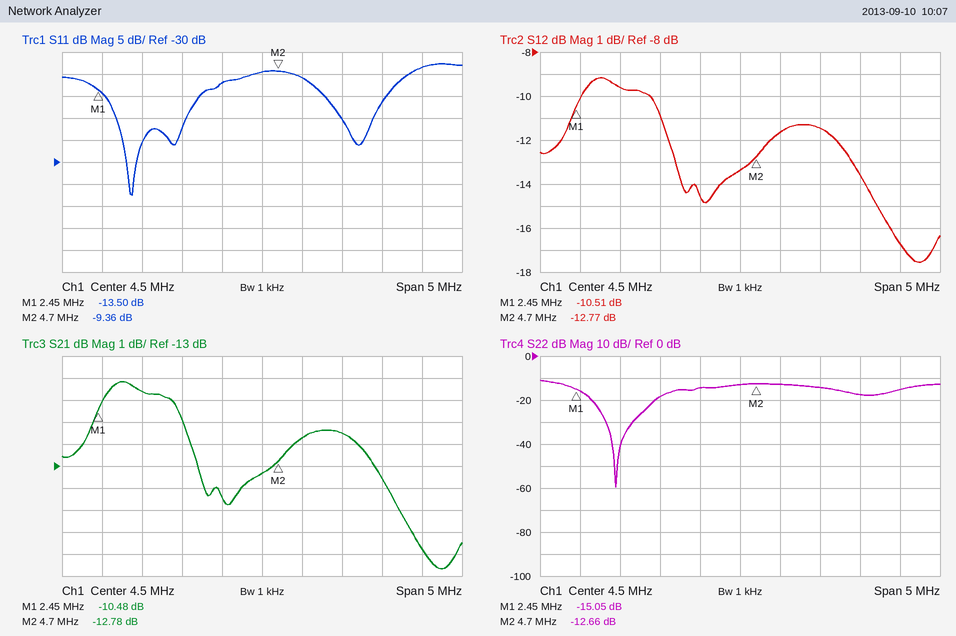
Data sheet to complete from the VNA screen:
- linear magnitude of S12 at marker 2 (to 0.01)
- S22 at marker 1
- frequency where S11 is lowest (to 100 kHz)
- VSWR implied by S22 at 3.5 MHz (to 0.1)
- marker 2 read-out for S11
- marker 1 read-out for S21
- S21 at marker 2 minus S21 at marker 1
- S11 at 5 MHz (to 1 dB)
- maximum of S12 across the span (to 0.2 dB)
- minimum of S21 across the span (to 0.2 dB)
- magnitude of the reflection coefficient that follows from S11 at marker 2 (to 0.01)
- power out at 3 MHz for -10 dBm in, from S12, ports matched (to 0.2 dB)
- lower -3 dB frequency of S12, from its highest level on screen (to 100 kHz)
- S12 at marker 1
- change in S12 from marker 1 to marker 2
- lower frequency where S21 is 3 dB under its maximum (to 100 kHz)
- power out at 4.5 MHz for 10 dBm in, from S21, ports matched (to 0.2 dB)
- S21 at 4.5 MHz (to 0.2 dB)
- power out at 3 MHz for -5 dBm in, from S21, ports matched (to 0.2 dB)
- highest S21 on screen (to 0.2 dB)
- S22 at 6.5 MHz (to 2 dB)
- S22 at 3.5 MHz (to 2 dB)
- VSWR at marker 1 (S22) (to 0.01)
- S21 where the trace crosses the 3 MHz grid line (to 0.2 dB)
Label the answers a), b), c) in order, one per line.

a) 0.23
b) -15.05 dB
c) 2.9 MHz
d) 1.3
e) -9.36 dB
f) -10.48 dB
g) -2.30 dB
h) -11 dB
i) -9.2 dB
j) -17.6 dB
k) 0.34
l) -19.6 dBm
m) 2.2 MHz
n) -10.51 dB
o) -2.26 dB
p) 2.2 MHz
q) -3.4 dBm
r) -13.4 dB
s) -14.6 dBm
t) -9.2 dB
u) -16 dB
v) -18 dB
w) 1.43
x) -9.6 dB
